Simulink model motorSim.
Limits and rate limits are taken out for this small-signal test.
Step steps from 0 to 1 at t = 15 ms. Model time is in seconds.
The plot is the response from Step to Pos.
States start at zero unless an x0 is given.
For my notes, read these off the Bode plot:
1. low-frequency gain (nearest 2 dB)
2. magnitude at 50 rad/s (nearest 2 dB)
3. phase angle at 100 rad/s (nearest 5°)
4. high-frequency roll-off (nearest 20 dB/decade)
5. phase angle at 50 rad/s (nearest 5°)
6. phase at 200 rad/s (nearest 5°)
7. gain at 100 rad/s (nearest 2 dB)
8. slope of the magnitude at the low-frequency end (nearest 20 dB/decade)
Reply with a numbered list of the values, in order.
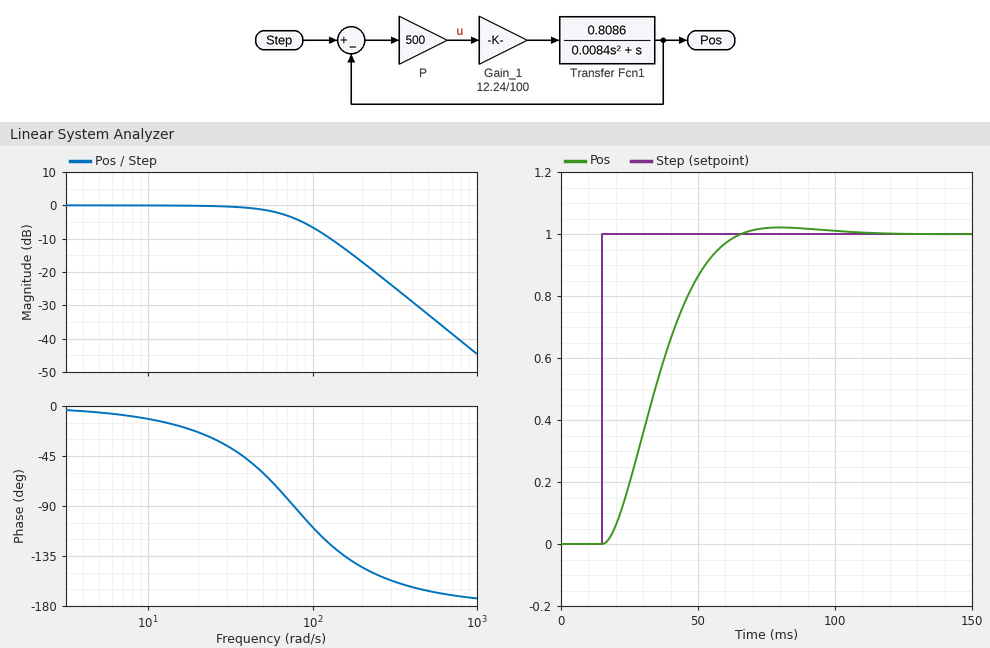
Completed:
1. 0 dB
2. -2 dB
3. -110°
4. -40 dB/decade
5. -60°
6. -145°
7. -6 dB
8. 0 dB/decade
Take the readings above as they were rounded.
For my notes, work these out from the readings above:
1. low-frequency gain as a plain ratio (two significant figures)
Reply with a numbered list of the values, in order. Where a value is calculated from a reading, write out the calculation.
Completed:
1. 10^(0 / 20) = 1.0
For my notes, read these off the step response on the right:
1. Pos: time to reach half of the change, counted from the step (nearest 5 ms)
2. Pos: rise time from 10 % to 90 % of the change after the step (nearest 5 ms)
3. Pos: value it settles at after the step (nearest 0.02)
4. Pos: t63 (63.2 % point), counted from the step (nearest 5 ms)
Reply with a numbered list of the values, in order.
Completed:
1. 20 ms
2. 30 ms
3. 1.00
4. 25 ms
